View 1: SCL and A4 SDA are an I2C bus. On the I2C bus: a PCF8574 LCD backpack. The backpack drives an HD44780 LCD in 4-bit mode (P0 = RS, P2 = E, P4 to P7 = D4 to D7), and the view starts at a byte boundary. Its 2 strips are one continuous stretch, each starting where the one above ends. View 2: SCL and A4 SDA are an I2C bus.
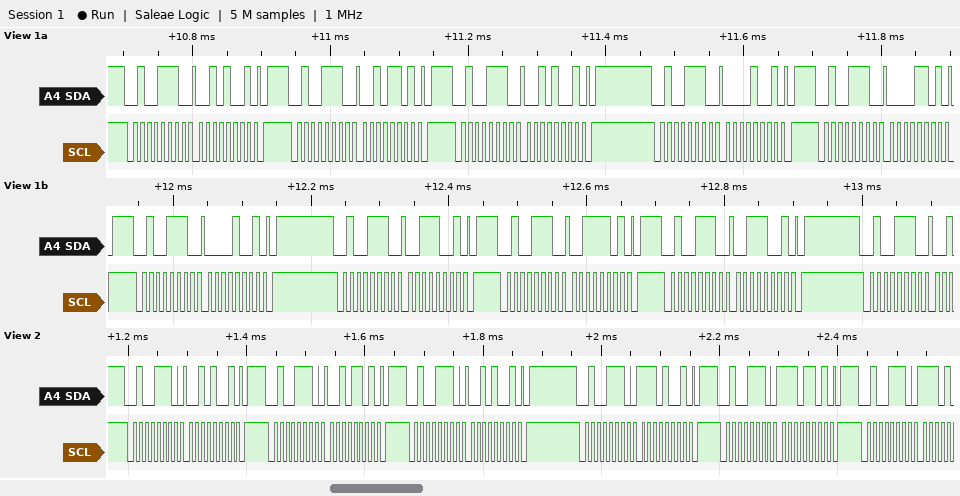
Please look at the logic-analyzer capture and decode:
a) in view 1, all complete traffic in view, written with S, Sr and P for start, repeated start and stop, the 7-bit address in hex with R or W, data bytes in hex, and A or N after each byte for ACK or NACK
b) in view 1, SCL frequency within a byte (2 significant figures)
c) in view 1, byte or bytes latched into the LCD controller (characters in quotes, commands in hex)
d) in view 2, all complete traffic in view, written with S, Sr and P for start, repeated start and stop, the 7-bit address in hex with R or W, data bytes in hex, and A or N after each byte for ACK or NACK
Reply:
S 27W A 29 A P S 27W A 2D A P S 27W A 29 A P S 27W A 09 A P S 27W A 0D A P S 27W A 09 A P S 27W A 39 A P S 27W A 3D A P S 27W A 39 A P S 27W A
100 kHz
' '
S 27W A 29 A P S 27W A 2D A P S 27W A 29 A P S 27W A E9 A P S 27W A ED A P S 27W A
